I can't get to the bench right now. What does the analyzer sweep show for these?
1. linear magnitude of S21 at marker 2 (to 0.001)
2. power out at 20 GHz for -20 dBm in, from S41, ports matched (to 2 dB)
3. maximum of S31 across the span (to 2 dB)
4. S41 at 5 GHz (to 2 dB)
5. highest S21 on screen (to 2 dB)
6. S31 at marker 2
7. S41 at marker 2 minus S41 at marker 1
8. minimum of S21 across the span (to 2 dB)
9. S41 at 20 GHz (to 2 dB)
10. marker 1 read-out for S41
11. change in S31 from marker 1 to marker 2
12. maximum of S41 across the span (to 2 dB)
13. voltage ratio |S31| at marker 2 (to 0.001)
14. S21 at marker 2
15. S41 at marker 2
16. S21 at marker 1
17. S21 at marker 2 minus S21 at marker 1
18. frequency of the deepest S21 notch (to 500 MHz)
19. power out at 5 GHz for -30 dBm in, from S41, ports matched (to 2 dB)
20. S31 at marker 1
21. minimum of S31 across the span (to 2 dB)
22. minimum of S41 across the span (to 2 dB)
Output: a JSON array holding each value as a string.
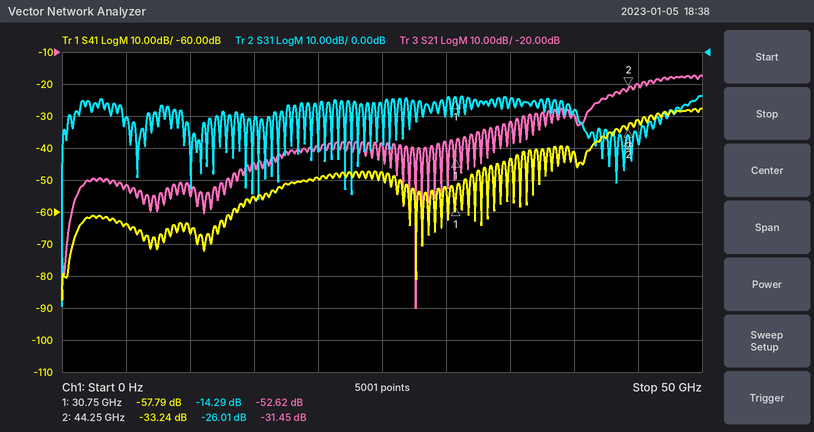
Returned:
["0.027", "-70 dBm", "-14 dB", "-64 dB", "-28 dB", "-26.01 dB", "24.55 dB", "-100 dB", "-50 dB", "-57.79 dB", "-11.72 dB", "-28 dB", "0.050", "-31.45 dB", "-33.24 dB", "-52.62 dB", "21.17 dB", "27.5 GHz", "-94 dBm", "-14.29 dB", "-80 dB", "-88 dB"]
